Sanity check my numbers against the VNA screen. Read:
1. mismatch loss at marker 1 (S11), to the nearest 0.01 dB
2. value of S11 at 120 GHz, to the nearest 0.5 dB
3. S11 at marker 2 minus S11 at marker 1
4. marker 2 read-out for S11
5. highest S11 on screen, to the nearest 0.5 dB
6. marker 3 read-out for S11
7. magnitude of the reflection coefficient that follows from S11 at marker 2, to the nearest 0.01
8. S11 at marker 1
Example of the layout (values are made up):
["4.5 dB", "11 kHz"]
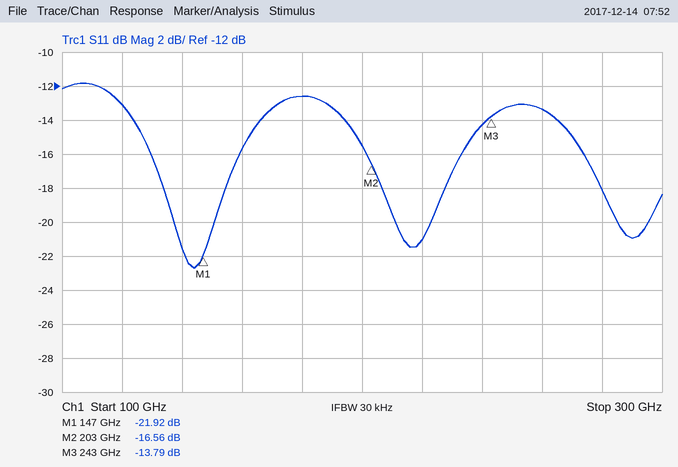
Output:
["0.03 dB", "-13.0 dB", "5.36 dB", "-16.56 dB", "-12.0 dB", "-13.79 dB", "0.15", "-21.92 dB"]
